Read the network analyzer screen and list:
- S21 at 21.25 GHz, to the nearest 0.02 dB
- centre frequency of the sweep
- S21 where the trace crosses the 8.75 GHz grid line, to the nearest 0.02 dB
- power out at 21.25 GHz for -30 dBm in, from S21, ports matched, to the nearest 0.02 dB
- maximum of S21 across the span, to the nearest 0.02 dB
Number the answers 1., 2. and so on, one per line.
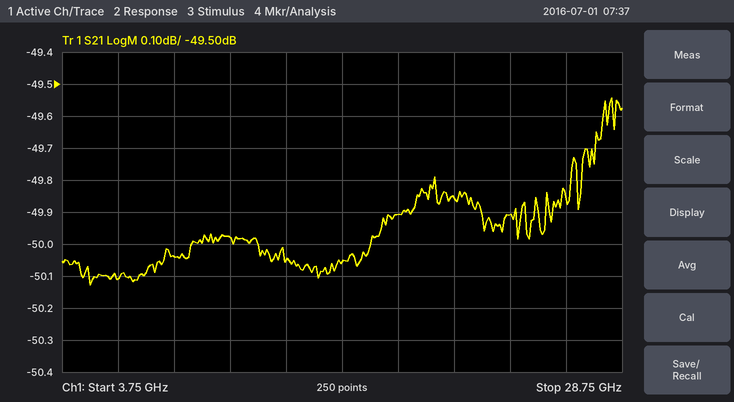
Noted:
1. -49.86 dB
2. 16.25 GHz
3. -50.04 dB
4. -79.86 dBm
5. -49.54 dB
